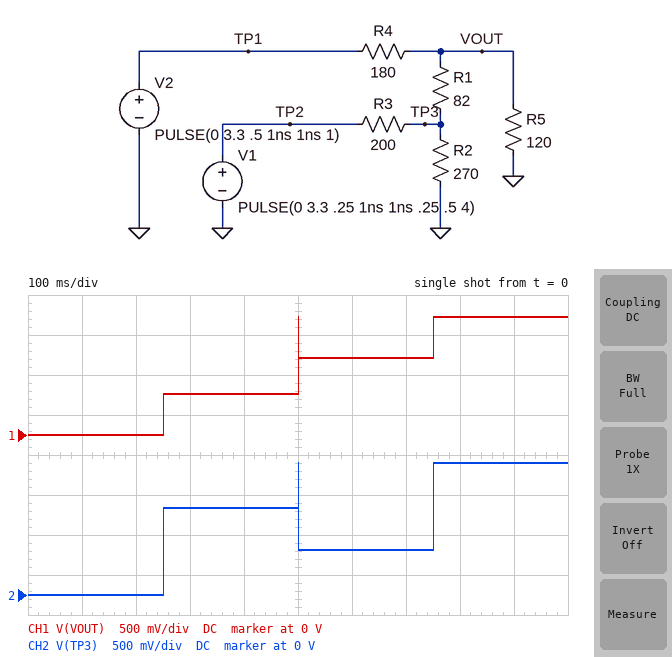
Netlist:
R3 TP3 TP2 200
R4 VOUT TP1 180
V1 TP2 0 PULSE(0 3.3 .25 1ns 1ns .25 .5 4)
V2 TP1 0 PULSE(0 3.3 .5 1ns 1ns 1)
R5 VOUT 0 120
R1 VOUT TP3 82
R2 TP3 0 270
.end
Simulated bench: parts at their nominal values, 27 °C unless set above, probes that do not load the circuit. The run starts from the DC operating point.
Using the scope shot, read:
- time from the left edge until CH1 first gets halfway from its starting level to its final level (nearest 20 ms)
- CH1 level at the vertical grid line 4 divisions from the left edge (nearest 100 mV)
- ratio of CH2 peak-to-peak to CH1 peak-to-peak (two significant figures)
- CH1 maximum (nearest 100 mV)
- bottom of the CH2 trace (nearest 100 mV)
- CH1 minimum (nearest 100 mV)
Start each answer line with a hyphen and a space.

- 500 ms
- 500 mV
- 1.1
- 1.5 V
- 0 V
- 0 V
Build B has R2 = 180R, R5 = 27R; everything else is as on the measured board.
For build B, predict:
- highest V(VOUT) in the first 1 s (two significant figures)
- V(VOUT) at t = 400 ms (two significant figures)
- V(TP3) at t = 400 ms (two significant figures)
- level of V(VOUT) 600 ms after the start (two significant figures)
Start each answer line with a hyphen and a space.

- 560 mV
- 180 mV
- 820 mV
- 380 mV
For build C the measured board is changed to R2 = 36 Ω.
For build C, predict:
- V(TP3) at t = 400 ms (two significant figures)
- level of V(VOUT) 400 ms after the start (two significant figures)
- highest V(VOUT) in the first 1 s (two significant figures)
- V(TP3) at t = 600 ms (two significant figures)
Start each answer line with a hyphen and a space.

- 420 mV
- 200 mV
- 1.0 V
- 220 mV
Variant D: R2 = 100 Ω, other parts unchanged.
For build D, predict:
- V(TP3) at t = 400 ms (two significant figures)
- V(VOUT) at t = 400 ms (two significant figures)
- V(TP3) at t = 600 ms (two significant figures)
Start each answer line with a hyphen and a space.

- 770 mV
- 360 mV
- 400 mV
